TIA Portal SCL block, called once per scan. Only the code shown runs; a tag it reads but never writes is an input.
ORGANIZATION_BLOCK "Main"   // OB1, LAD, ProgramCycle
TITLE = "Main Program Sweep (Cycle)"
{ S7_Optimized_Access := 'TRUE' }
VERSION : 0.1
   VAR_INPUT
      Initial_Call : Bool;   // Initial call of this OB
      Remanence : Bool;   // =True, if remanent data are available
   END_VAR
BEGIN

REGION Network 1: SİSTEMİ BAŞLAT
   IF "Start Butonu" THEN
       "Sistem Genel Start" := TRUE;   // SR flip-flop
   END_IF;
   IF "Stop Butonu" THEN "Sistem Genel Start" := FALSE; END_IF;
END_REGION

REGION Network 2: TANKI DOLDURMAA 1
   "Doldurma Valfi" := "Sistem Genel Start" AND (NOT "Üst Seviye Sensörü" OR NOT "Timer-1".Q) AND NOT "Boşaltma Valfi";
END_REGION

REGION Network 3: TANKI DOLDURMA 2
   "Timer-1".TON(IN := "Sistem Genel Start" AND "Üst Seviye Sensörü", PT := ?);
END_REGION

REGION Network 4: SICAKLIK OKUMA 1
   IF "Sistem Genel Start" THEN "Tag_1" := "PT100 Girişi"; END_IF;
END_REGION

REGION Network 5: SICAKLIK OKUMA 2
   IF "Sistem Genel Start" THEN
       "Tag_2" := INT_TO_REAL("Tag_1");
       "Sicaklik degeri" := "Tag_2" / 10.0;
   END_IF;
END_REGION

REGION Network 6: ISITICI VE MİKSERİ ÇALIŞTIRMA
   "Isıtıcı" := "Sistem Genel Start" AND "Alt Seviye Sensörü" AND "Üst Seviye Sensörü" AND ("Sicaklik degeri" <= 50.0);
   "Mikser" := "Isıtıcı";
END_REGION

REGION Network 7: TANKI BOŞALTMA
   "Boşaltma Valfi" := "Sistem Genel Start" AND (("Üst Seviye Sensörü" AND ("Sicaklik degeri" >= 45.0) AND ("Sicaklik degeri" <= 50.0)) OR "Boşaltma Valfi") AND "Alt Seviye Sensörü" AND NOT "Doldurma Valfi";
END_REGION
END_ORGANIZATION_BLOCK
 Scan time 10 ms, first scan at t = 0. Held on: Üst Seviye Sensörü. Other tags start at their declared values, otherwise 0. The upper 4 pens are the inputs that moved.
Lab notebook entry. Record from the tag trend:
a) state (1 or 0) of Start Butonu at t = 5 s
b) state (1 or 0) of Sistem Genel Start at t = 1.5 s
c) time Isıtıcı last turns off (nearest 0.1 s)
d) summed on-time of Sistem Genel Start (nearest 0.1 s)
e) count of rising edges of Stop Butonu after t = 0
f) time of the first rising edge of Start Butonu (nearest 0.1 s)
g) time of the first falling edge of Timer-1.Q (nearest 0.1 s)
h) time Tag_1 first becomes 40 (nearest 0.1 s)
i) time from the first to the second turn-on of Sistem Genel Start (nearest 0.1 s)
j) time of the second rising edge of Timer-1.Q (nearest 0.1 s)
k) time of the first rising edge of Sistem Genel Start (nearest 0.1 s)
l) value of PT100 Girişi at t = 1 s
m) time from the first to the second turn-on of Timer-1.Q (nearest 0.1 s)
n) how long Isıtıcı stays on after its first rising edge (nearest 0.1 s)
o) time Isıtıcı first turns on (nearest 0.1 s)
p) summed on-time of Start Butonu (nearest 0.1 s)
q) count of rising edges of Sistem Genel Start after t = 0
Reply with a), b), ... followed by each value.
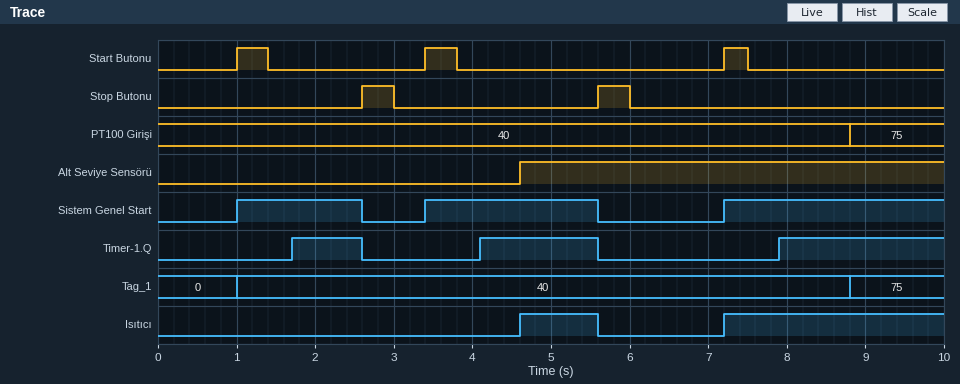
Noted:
a) 0
b) 1
c) 5.6 s
d) 6.6 s
e) 2
f) 1.0 s
g) 2.6 s
h) 1.0 s
i) 2.4 s
j) 4.1 s
k) 1.0 s
l) 40
m) 2.4 s
n) 1.0 s
o) 4.6 s
p) 1.1 s
q) 3
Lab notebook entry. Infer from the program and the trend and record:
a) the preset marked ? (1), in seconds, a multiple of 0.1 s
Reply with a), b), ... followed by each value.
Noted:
a) 0.7 s
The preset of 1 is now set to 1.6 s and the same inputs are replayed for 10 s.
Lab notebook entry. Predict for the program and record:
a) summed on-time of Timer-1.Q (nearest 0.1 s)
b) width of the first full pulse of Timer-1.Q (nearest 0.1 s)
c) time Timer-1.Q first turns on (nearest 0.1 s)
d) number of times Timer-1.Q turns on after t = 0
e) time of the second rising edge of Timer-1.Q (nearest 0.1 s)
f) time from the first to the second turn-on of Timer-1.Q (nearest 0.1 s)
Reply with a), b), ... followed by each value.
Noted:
a) 1.8 s
b) 0.6 s
c) 5.0 s
d) 2
e) 8.8 s
f) 3.8 s
